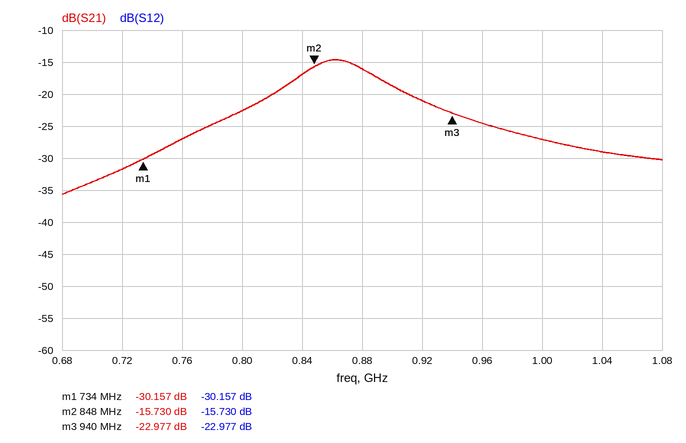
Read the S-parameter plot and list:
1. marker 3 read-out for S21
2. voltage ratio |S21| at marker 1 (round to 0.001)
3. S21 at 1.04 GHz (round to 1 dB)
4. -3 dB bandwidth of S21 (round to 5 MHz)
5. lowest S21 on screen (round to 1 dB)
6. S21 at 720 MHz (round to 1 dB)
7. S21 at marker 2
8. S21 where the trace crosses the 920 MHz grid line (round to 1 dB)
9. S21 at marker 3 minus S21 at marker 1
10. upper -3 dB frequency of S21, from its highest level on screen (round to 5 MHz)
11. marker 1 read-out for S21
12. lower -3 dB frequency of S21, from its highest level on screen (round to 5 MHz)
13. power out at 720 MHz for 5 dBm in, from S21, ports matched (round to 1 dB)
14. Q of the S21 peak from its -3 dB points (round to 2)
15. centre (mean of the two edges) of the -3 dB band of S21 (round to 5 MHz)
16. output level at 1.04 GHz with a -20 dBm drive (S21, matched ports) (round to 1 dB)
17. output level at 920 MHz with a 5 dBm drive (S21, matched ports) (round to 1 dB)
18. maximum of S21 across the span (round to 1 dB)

-22.977 dB
0.031
-29 dB
55 MHz
-36 dB
-32 dB
-15.730 dB
-21 dB
7.180 dB
890 MHz
-30.157 dB
835 MHz
-27 dBm
16
865 MHz
-49 dBm
-16 dBm
-15 dB
